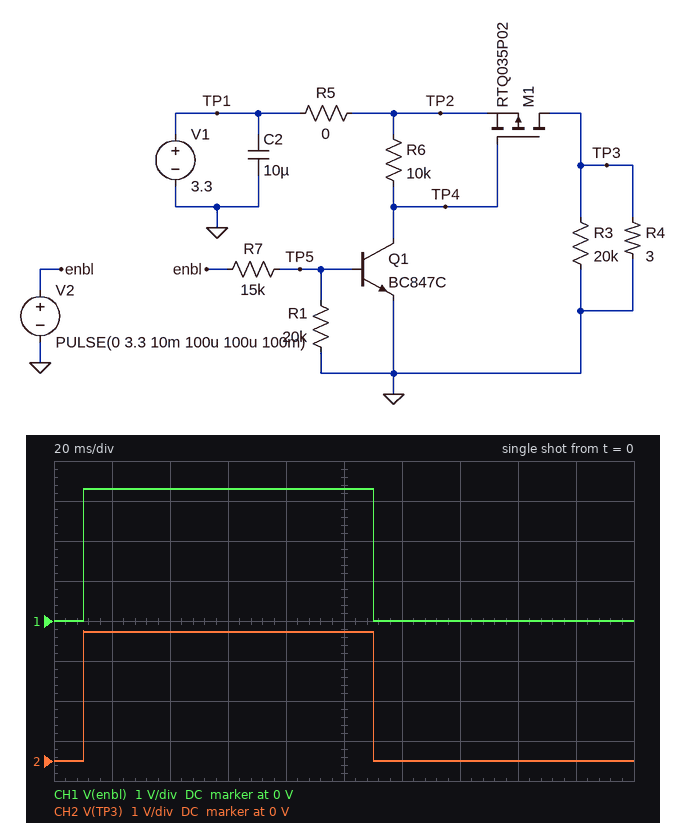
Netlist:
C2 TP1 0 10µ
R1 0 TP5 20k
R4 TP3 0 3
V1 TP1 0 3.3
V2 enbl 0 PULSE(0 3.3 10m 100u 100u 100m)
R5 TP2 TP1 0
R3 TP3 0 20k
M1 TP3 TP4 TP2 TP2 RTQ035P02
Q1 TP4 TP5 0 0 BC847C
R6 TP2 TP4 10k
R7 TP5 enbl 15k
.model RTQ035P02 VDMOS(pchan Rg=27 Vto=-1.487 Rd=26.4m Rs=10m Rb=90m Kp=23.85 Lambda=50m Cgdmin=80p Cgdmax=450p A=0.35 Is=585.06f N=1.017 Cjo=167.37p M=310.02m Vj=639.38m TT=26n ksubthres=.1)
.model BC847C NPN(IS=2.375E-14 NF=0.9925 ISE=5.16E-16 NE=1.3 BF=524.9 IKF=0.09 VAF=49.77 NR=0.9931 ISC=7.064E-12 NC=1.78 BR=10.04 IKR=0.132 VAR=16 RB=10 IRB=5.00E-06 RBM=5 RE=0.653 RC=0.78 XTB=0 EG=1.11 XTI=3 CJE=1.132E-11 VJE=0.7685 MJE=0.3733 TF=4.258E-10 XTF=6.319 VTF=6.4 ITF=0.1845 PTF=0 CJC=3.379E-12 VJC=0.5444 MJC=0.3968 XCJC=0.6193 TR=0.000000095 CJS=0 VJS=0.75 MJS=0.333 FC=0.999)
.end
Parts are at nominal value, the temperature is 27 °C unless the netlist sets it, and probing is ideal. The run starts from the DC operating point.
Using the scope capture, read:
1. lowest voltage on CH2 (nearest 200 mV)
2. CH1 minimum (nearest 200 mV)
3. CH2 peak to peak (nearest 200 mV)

0 V
0 V
3.2 V
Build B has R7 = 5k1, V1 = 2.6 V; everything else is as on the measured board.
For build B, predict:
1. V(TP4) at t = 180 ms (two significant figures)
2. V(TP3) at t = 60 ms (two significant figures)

2.6 V
2.5 V
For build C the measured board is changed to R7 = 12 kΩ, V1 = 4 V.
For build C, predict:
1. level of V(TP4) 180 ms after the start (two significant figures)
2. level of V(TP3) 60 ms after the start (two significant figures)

4.0 V
3.9 V
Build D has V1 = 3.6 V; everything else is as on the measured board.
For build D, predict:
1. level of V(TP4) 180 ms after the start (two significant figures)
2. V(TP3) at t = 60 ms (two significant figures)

3.6 V
3.5 V
